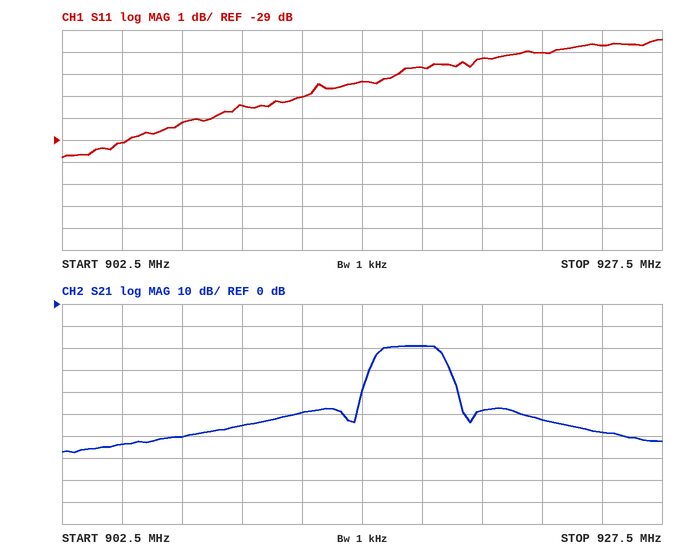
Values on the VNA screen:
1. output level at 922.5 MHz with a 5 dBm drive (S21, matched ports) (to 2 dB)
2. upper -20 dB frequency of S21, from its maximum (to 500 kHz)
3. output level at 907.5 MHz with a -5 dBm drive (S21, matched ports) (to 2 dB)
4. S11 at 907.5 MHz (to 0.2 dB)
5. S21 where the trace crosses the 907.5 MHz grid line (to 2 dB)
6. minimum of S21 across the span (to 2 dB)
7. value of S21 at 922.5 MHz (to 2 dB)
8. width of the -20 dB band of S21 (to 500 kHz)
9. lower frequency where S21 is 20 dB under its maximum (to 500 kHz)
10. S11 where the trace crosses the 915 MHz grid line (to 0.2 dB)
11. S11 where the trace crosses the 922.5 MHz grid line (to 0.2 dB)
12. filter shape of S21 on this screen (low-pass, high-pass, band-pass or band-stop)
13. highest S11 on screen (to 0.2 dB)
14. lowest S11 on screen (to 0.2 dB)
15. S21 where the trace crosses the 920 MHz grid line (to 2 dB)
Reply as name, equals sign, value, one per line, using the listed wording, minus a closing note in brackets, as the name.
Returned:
output level at 922.5 MHz with a 5 dBm drive (S21, matched ports) = -48 dBm
upper -20 dB frequency of S21, from its maximum = 919.0 MHz
output level at 907.5 MHz with a -5 dBm drive (S21, matched ports) = -66 dBm
S11 at 907.5 MHz = -28.2 dB
S21 where the trace crosses the 907.5 MHz grid line = -60 dB
minimum of S21 across the span = -68 dB
value of S21 at 922.5 MHz = -52 dB
width of the -20 dB band of S21 = 4.0 MHz
lower frequency where S21 is 20 dB under its maximum = 915.0 MHz
S11 where the trace crosses the 915 MHz grid line = -26.4 dB
S11 where the trace crosses the 922.5 MHz grid line = -25.0 dB
filter shape of S21 on this screen = band-pass
highest S11 on screen = -24.4 dB
lowest S11 on screen = -29.8 dB
S21 where the trace crosses the 920 MHz grid line = -48 dB
